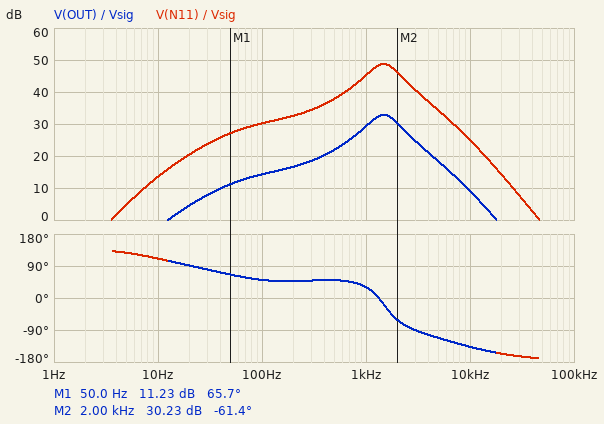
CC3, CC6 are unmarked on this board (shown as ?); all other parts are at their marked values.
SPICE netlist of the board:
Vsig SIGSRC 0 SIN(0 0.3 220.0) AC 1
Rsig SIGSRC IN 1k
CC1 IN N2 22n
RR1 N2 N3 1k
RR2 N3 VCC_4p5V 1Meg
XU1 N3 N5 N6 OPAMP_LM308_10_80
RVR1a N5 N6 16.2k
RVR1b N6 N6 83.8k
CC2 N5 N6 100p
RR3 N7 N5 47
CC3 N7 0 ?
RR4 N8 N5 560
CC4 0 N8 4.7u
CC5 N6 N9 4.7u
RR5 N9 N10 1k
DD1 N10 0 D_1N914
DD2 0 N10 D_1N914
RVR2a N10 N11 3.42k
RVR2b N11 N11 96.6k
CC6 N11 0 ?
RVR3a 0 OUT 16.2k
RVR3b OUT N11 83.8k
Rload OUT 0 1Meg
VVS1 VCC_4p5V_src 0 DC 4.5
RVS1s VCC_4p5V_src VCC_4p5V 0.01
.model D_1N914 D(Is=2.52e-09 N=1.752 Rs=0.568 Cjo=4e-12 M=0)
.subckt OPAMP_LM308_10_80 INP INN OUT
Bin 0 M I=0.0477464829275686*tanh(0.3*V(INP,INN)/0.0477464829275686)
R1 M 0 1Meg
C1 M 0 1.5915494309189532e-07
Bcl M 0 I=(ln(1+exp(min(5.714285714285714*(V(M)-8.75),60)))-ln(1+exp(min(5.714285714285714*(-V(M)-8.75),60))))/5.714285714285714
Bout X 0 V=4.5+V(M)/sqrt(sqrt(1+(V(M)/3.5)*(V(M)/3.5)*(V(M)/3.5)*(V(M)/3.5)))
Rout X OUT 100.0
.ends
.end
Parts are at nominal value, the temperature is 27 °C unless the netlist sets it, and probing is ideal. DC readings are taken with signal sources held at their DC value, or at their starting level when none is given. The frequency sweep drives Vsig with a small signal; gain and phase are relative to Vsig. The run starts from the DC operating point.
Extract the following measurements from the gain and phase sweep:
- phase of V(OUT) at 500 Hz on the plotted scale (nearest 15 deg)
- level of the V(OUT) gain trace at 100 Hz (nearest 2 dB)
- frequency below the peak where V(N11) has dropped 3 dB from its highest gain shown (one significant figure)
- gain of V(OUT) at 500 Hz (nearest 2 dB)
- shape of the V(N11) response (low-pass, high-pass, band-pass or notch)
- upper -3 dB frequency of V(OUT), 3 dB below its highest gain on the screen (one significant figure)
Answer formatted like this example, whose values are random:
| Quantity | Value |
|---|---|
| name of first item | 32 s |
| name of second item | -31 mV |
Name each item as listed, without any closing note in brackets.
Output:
| Quantity | Value |
|---|---|
| phase of V(OUT) at 500 Hz on the plotted scale | 45 deg |
| level of the V(OUT) gain trace at 100 Hz | 14 dB |
| frequency below the peak where V(N11) has dropped 3 dB from its highest gain shown | 1 kHz |
| gain of V(OUT) at 500 Hz | 22 dB |
| shape of the V(N11) response | band-pass |
| upper -3 dB frequency of V(OUT), 3 dB below its highest gain on the screen | 2 kHz |
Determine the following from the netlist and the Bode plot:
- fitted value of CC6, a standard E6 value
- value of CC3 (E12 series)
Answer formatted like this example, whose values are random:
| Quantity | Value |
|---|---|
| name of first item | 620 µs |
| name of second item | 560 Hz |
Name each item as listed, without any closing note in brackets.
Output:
| Quantity | Value |
|---|---|
| fitted value of CC6, a standard E6 value | 4.7 nF |
| value of CC3 | 1.2 µF |
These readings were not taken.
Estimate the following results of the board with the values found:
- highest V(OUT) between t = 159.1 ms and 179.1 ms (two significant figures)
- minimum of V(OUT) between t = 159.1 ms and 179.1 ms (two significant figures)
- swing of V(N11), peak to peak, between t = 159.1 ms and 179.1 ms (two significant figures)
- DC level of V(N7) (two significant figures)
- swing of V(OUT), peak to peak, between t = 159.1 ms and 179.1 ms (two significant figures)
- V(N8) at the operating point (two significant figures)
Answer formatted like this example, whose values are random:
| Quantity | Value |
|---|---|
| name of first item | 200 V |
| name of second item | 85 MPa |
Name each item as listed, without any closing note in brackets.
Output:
| Quantity | Value |
|---|---|
| highest V(OUT) between t = 159.1 ms and 179.1 ms | 98 mV |
| minimum of V(OUT) between t = 159.1 ms and 179.1 ms | -98 mV |
| swing of V(N11), peak to peak, between t = 159.1 ms and 179.1 ms | 1.2 V |
| DC level of V(N7) | 4.5 V |
| swing of V(OUT), peak to peak, between t = 159.1 ms and 179.1 ms | 200 mV |
| V(N8) at the operating point | 4.5 V |
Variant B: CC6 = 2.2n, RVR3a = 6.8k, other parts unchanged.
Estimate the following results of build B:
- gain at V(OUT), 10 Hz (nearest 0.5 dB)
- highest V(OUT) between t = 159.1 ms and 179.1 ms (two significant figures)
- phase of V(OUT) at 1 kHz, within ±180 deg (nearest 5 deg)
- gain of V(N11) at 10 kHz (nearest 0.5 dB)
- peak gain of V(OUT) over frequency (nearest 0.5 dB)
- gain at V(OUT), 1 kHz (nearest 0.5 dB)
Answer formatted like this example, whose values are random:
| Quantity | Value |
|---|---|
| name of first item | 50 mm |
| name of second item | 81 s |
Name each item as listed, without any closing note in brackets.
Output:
| Quantity | Value |
|---|---|
| gain at V(OUT), 10 Hz | -9.0 dB |
| highest V(OUT) between t = 159.1 ms and 179.1 ms | 46 mV |
| phase of V(OUT) at 1 kHz, within ±180 deg | 35 deg |
| gain of V(N11) at 10 kHz | 28.0 dB |
| peak gain of V(OUT) over frequency | 26.5 dB |
| gain at V(OUT), 1 kHz | 22.5 dB |
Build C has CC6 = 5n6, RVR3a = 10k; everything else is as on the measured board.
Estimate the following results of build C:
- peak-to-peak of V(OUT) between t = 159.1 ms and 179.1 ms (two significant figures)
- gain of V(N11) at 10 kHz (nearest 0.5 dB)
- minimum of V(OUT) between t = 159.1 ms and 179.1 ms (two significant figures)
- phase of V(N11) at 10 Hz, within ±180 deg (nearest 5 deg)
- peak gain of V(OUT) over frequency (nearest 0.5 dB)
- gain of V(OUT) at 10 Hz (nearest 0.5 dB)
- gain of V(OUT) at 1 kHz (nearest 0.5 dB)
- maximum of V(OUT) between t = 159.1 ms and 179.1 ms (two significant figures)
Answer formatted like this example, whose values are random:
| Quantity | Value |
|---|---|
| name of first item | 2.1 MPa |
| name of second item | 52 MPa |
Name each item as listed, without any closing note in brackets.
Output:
| Quantity | Value |
|---|---|
| peak-to-peak of V(OUT) between t = 159.1 ms and 179.1 ms | 130 mV |
| gain of V(N11) at 10 kHz | 24.0 dB |
| minimum of V(OUT) between t = 159.1 ms and 179.1 ms | -65 mV |
| phase of V(N11) at 10 Hz, within ±180 deg | 110 deg |
| peak gain of V(OUT) over frequency | 29.0 dB |
| gain of V(OUT) at 10 Hz | -6.0 dB |
| gain of V(OUT) at 1 kHz | 25.5 dB |
| maximum of V(OUT) between t = 159.1 ms and 179.1 ms | 65 mV |
